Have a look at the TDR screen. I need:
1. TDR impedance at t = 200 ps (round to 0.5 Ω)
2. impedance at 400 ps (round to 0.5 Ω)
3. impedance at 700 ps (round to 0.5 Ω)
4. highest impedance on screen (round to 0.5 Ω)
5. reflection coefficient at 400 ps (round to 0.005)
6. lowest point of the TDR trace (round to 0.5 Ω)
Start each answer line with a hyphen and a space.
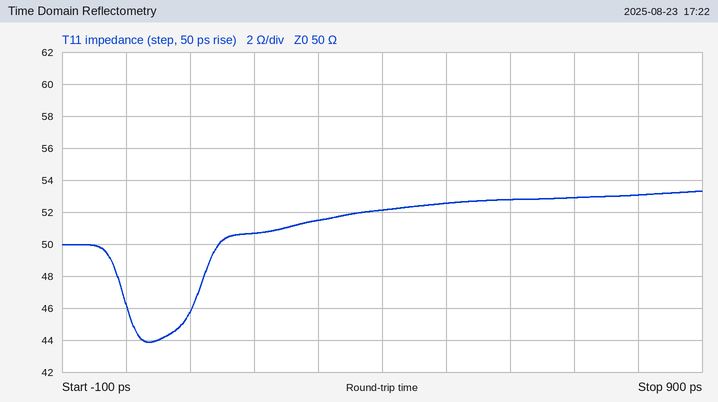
- 50.5 Ω
- 52.0 Ω
- 53.0 Ω
- 53.5 Ω
- +0.020
- 44.0 Ω
